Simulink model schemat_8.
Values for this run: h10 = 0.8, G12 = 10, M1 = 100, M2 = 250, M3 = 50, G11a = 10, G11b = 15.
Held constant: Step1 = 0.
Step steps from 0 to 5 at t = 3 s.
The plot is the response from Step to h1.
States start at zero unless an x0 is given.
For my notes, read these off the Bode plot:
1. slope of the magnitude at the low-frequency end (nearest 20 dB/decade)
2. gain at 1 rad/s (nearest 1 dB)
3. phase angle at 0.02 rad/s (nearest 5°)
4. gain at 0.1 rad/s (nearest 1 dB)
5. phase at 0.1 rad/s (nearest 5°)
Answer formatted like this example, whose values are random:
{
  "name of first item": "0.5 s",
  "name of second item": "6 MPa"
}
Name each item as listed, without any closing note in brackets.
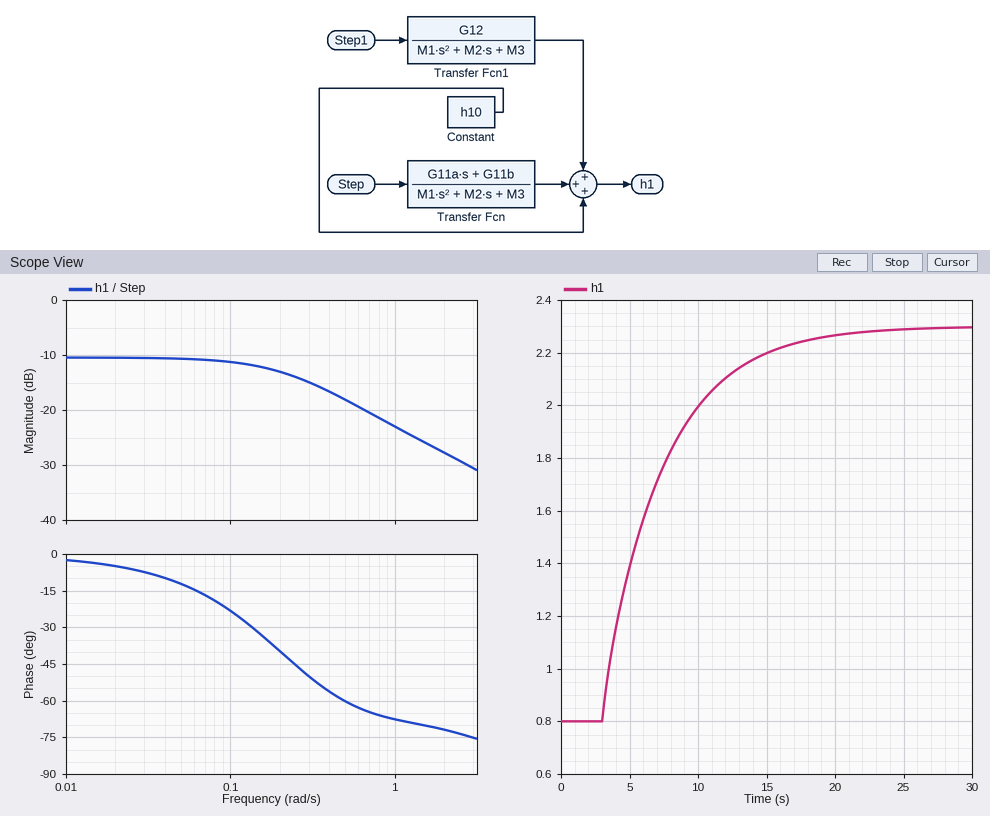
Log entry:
{
  "slope of the magnitude at the low-frequency end": "0 dB/decade",
  "gain at 1 rad/s": "-23 dB",
  "phase angle at 0.02 rad/s": "-5°",
  "gain at 0.1 rad/s": "-11 dB",
  "phase at 0.1 rad/s": "-25°"
}
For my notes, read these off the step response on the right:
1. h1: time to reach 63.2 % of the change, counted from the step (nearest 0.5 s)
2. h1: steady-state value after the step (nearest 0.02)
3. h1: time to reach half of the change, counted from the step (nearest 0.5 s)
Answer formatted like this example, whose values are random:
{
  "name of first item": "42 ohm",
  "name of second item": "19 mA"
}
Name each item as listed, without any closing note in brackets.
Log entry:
{
  "h1: time to reach 63.2 % of the change, counted from the step": "4.5 s",
  "h1: steady-state value after the step": "2.30",
  "h1: time to reach half of the change, counted from the step": "3.0 s"
}
